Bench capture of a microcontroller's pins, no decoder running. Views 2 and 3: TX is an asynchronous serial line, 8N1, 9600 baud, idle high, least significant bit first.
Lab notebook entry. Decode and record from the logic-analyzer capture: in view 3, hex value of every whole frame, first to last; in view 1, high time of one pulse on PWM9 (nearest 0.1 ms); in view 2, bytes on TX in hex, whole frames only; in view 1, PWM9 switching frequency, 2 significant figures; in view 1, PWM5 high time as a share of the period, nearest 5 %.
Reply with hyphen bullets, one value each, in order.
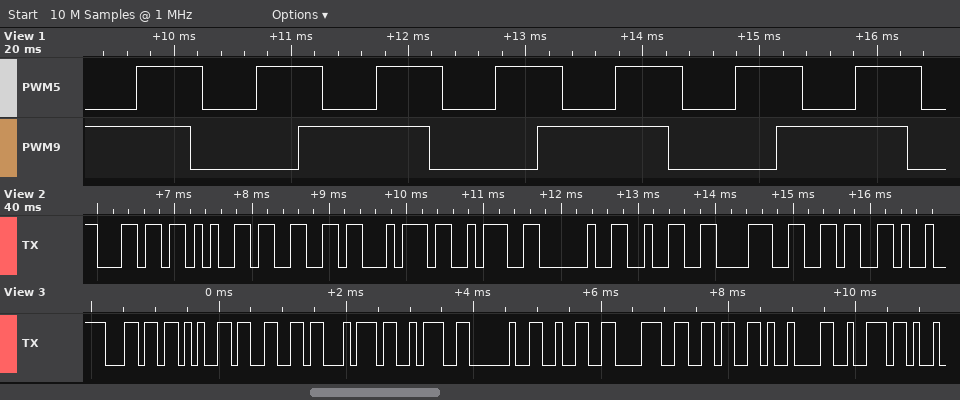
- 6C 65 66 74 3A 20 32 38 36 09 72
- 1.1 ms
- 6C 65 66 74 3A 20 32 38 36
- 490 Hz
- 55 %
